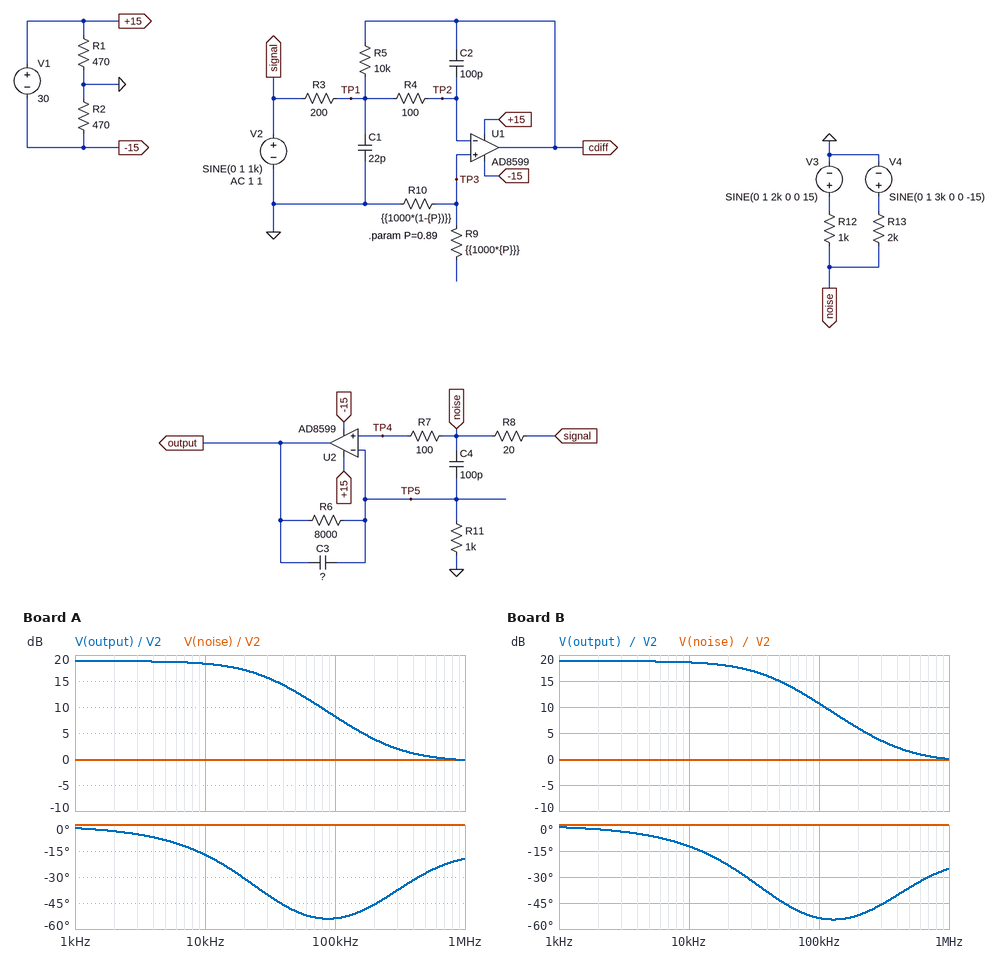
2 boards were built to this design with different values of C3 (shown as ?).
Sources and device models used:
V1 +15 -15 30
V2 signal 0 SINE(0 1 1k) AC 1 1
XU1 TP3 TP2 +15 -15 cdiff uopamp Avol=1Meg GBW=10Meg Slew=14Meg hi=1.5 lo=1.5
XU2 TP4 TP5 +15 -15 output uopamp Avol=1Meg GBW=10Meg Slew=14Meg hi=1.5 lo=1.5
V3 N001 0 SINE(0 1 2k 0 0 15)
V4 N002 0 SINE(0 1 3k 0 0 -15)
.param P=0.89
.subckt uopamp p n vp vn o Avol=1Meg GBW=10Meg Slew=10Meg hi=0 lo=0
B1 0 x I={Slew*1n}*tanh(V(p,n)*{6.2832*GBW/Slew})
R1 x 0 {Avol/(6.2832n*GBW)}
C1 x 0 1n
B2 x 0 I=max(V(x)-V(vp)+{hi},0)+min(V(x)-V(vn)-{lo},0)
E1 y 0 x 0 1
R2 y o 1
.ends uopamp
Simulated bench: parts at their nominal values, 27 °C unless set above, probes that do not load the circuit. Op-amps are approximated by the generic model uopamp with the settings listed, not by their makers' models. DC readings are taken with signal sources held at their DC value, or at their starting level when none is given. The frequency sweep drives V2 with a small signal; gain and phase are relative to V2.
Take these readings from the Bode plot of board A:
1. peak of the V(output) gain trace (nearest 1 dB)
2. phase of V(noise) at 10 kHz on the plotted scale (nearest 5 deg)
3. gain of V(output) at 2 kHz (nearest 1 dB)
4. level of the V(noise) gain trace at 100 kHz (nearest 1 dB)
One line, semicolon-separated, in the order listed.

19 dB; 0 deg; 19 dB; 0 dB
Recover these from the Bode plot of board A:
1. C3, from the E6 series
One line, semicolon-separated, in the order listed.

680 pF
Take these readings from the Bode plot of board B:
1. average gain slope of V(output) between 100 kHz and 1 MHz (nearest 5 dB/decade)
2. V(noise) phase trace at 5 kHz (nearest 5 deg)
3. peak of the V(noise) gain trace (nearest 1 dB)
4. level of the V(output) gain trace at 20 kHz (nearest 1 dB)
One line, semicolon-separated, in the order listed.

-10 dB/decade; 0 deg; 0 dB; 18 dB
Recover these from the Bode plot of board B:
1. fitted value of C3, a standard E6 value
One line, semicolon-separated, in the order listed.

470 pF
